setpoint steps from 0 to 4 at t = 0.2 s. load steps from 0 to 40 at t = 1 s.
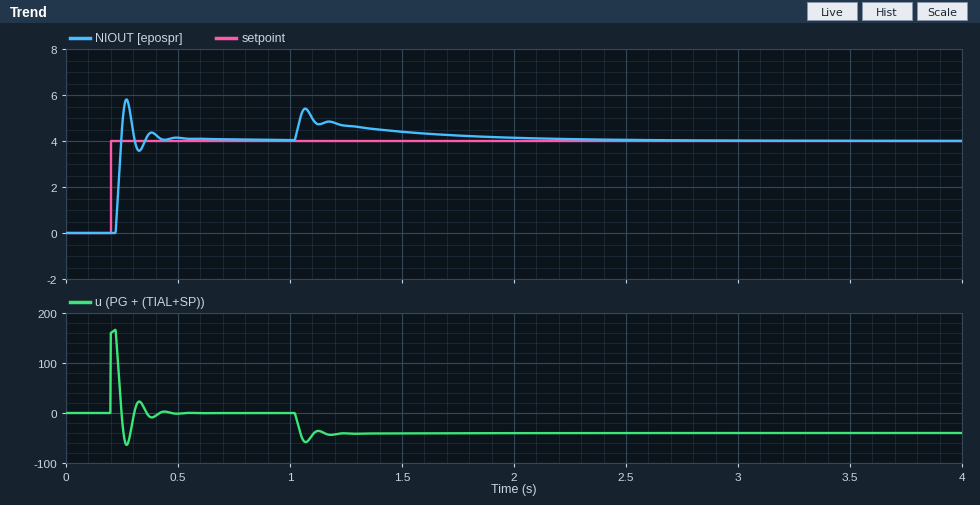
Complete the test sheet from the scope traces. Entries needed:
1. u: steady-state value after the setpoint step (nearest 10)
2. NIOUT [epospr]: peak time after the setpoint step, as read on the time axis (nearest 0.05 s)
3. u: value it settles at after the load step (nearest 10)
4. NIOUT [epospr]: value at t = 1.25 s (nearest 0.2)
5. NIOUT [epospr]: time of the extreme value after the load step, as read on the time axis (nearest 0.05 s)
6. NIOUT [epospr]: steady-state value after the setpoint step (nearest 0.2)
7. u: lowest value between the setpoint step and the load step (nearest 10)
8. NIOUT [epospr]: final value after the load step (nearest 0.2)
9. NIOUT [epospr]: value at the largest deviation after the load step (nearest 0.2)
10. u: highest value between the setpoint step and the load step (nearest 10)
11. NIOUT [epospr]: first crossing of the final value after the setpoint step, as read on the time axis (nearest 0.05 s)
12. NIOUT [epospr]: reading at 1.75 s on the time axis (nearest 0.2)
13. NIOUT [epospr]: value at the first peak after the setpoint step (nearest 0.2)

0
0.25 s
-40
4.6
1.05 s
4.0
-60
4.0
5.4
170
0.25 s
4.2
5.8
